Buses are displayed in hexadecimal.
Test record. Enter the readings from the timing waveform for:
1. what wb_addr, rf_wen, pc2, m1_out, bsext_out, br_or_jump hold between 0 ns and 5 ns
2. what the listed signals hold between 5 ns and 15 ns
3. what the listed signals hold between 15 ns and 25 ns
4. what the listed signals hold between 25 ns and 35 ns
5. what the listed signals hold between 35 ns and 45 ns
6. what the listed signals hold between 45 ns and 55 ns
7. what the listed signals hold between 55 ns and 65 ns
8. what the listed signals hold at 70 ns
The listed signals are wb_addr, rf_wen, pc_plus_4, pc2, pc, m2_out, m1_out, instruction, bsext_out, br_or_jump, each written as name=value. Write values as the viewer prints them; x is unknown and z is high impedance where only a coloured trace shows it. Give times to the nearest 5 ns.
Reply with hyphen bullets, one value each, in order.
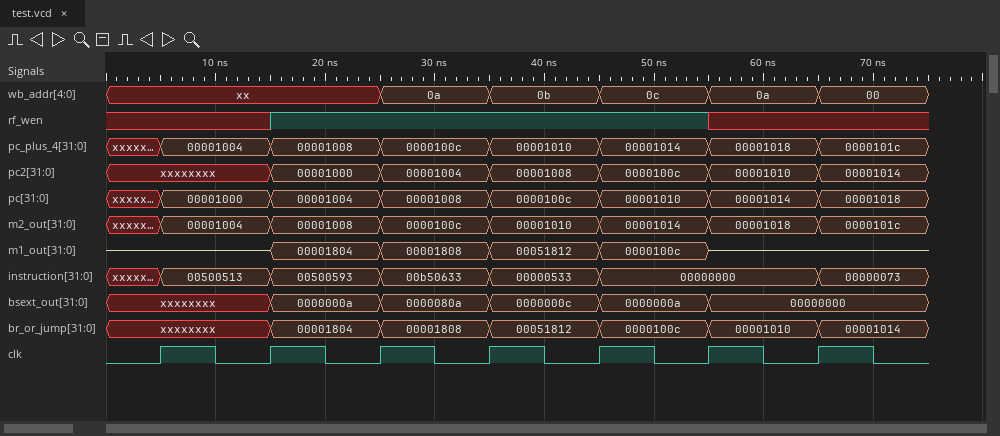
- wb_addr=xx, rf_wen=x, pc2=xxxxxxxx, m1_out=z, bsext_out=xxxxxxxx, br_or_jump=xxxxxxxx
- wb_addr=xx, rf_wen=x, pc_plus_4=00001004, pc2=xxxxxxxx, pc=00001000, m2_out=00001004, m1_out=z, instruction=00500513, bsext_out=xxxxxxxx, br_or_jump=xxxxxxxx
- wb_addr=xx, rf_wen=1, pc_plus_4=00001008, pc2=00001000, pc=00001004, m2_out=00001008, m1_out=00001804, instruction=00500593, bsext_out=0000000a, br_or_jump=00001804
- wb_addr=0a, rf_wen=1, pc_plus_4=0000100c, pc2=00001004, pc=00001008, m2_out=0000100c, m1_out=00001808, instruction=00b50633, bsext_out=0000080a, br_or_jump=00001808
- wb_addr=0b, rf_wen=1, pc_plus_4=00001010, pc2=00001008, pc=0000100c, m2_out=00001010, m1_out=00051812, instruction=00000533, bsext_out=0000000c, br_or_jump=00051812
- wb_addr=0c, rf_wen=1, pc_plus_4=00001014, pc2=0000100c, pc=00001010, m2_out=00001014, m1_out=0000100c, instruction=00000000, bsext_out=0000000a, br_or_jump=0000100c
- wb_addr=0a, rf_wen=x, pc_plus_4=00001018, pc2=00001010, pc=00001014, m2_out=00001018, m1_out=z, instruction=00000000, bsext_out=00000000, br_or_jump=00001010
- wb_addr=00, rf_wen=x, pc_plus_4=0000101c, pc2=00001014, pc=00001018, m2_out=0000101c, m1_out=z, instruction=00000073, bsext_out=00000000, br_or_jump=00001014
